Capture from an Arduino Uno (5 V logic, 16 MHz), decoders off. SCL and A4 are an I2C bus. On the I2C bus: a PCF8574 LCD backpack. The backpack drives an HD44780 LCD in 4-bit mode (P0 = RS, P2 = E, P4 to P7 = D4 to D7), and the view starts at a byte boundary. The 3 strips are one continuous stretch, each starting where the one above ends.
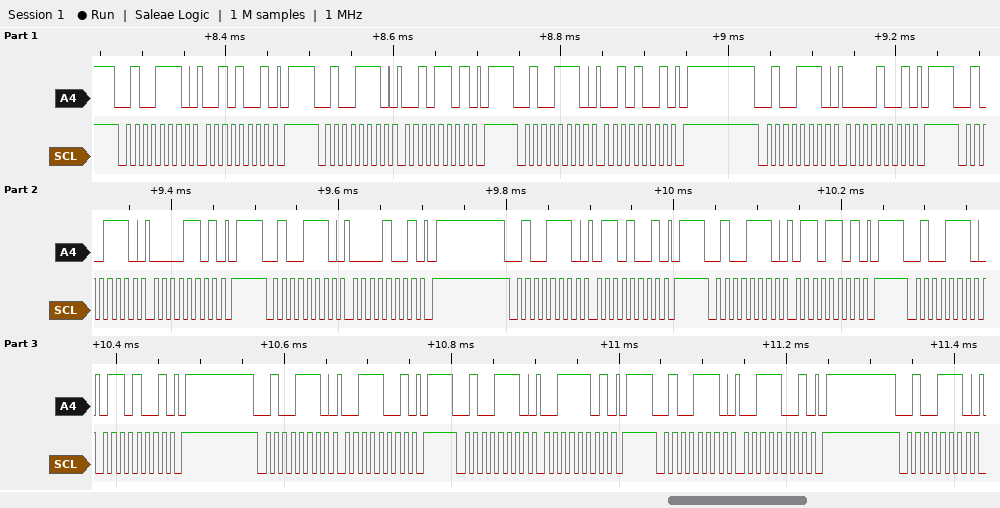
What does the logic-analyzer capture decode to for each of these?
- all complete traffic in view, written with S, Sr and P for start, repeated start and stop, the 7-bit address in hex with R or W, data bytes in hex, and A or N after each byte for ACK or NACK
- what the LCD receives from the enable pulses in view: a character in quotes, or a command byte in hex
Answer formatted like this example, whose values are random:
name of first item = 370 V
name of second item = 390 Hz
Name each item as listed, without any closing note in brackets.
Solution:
all complete traffic in view, written with S, Sr and P for start, repeated start and stop, the 7-bit address in hex with R or W, data bytes in hex, and A or N after each byte for ACK or NACK = S 27W A 29 A P S 27W A 2D A P S 27W A 29 A P S 27W A 09 A P S 27W A 0D A P S 27W A 09 A P S 27W A 69 A P S 27W A 6D A P S 27W A 69 A P S 27W A 39 A P S 27W A 3D A P S 27W A 39 A P S 27W A
what the LCD receives from the enable pulses in view: a character in quotes, or a command byte in hex = ' ' 'c'
